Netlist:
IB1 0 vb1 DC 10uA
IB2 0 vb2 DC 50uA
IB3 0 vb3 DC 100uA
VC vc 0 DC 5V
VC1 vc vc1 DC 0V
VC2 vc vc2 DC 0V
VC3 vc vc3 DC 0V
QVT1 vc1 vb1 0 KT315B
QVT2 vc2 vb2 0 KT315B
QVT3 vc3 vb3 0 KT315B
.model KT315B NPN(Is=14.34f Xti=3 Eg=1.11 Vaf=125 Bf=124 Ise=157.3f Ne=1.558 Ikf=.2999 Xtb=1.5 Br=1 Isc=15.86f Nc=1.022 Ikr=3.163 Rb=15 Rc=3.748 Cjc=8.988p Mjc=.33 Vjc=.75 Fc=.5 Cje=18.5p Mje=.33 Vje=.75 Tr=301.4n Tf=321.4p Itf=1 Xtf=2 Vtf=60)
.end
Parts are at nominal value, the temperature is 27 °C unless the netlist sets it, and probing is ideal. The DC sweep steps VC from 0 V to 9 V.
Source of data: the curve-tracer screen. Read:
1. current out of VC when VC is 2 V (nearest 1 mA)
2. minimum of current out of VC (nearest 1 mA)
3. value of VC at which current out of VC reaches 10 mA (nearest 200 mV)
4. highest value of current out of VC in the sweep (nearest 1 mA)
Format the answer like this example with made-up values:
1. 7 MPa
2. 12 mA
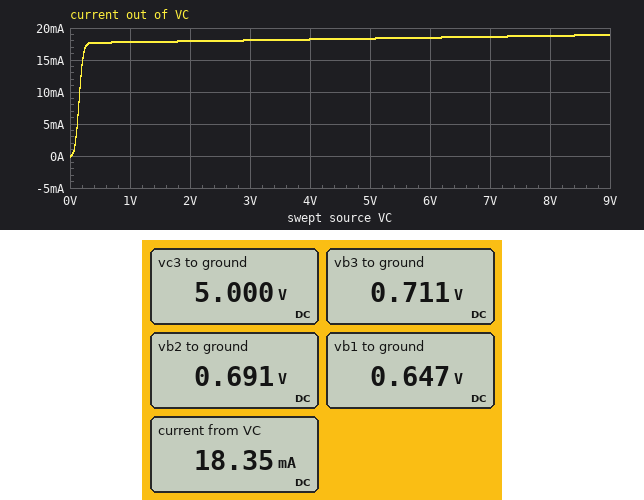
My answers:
1. 18 mA
2. 0 A
3. 200 mV
4. 19 mA
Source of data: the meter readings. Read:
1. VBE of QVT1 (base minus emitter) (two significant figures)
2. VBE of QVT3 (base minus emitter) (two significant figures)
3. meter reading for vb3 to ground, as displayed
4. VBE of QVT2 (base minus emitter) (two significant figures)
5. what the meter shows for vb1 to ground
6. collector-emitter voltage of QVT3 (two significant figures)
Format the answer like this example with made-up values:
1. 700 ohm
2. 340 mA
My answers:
1. 650 mV
2. 710 mV
3. 0.711 V
4. 690 mV
5. 0.647 V
6. 5.0 V
